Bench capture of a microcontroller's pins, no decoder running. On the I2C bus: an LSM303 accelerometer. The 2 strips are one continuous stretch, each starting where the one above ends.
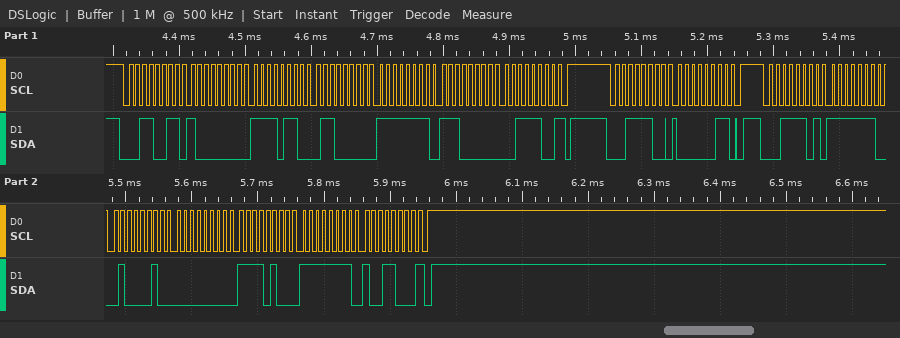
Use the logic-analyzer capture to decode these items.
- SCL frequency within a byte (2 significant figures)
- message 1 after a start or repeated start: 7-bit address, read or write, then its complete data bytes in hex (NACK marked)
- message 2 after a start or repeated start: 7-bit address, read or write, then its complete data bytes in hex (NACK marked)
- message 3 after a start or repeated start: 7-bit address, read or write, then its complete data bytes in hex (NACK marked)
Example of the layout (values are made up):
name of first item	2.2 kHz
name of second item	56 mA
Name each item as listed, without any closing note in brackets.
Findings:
SCL frequency within a byte	100 kHz
message 1 after a start or repeated start: 7-bit address, read or write, then its complete data bytes in hex	0x19 read: 80 F6 60 FF E0 3C NACK
message 2 after a start or repeated start: 7-bit address, read or write, then its complete data bytes in hex	0x1E write: 03
message 3 after a start or repeated start: 7-bit address, read or write, then its complete data bytes in hex	0x1E read: FE 42 00 F4 FF 98 NACK
